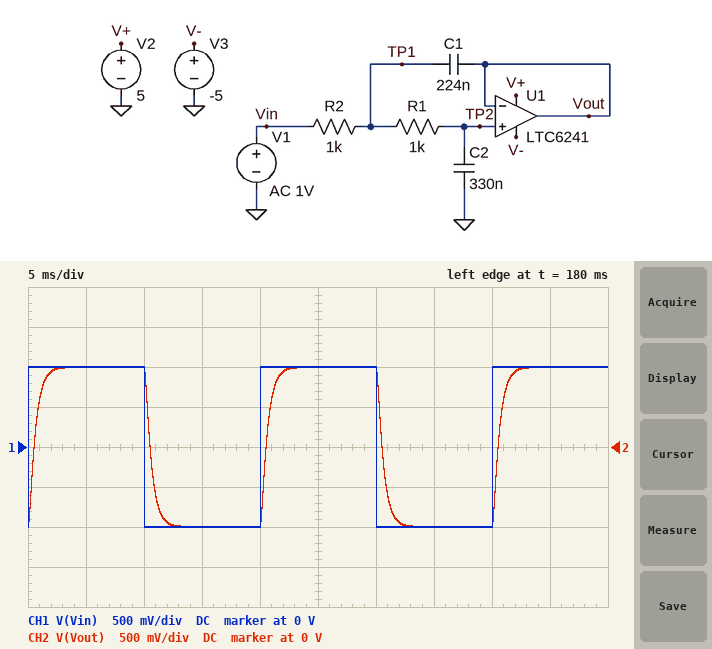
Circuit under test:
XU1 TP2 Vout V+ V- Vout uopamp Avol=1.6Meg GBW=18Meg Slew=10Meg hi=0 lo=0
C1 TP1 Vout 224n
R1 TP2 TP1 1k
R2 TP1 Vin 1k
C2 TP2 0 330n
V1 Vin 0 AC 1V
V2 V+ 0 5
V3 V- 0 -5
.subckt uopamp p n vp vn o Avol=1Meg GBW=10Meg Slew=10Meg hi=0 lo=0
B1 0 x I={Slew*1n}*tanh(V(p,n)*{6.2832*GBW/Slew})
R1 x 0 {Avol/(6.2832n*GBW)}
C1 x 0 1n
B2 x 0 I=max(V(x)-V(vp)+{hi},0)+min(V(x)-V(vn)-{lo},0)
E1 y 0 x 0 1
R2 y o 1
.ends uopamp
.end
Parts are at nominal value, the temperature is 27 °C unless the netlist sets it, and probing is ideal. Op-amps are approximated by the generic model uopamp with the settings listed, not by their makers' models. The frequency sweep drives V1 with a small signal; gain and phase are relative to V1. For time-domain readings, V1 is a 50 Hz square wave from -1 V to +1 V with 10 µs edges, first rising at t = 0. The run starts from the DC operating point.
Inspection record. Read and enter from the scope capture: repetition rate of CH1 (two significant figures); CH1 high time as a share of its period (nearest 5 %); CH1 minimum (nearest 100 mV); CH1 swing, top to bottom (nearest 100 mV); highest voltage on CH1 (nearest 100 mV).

50 Hz
50 %
-1.0 V
2.0 V
1.0 V
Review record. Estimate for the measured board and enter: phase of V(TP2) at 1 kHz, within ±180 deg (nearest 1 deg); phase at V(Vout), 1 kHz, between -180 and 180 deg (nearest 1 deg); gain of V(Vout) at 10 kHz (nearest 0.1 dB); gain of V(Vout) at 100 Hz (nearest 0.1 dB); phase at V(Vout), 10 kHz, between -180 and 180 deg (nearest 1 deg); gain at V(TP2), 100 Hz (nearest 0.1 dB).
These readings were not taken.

-115 deg
-115 deg
-49.4 dB
-0.5 dB
-172 deg
-0.5 dB
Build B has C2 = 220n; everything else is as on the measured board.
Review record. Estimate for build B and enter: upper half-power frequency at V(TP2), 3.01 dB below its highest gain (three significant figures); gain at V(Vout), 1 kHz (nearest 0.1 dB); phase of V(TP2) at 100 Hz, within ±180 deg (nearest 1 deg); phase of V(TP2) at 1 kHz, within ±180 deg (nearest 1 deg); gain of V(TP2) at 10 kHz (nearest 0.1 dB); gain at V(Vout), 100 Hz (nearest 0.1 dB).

467 Hz
-9.3 dB
-16 deg
-109 deg
-45.8 dB
-0.2 dB
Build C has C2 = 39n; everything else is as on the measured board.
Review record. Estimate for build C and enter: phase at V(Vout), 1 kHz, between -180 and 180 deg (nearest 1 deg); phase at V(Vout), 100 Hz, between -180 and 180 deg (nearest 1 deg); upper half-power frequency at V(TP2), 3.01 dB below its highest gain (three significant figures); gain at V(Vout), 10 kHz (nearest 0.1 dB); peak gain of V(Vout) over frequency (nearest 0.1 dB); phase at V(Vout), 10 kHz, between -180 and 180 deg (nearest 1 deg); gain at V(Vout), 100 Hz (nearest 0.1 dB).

-37 deg
-3 deg
2.02 kHz
-30.6 dB
2.4 dB
-172 deg
0 dB
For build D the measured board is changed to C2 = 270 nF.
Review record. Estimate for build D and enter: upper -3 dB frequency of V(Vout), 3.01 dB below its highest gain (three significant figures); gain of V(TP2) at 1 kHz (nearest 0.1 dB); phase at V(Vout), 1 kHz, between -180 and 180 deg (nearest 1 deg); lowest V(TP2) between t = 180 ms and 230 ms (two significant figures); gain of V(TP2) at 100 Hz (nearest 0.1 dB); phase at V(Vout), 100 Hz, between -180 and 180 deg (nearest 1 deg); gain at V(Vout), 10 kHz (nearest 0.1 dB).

365 Hz
-11.3 dB
-112 deg
-1.0 V
-0.3 dB
-19 deg
-47.6 dB
